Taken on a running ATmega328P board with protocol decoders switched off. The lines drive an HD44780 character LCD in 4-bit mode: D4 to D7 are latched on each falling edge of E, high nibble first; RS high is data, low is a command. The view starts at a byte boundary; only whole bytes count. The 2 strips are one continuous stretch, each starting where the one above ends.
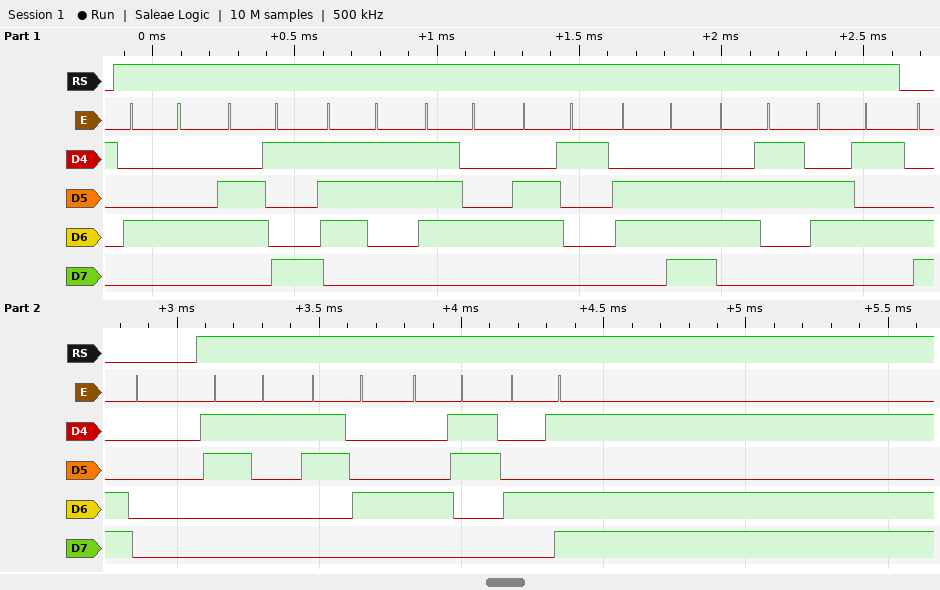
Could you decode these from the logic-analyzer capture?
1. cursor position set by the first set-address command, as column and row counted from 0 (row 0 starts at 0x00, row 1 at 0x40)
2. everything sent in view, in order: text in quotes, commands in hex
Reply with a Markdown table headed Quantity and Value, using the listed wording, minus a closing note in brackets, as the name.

| Quantity | Value |
|---|---|
| cursor position set by the first set-address command, as column and row counted from 0 | column 0, row 1 |
| everything sent in view, in order: text in quotes, commands in hex | "Distance" 0xC0 "14CM" |
